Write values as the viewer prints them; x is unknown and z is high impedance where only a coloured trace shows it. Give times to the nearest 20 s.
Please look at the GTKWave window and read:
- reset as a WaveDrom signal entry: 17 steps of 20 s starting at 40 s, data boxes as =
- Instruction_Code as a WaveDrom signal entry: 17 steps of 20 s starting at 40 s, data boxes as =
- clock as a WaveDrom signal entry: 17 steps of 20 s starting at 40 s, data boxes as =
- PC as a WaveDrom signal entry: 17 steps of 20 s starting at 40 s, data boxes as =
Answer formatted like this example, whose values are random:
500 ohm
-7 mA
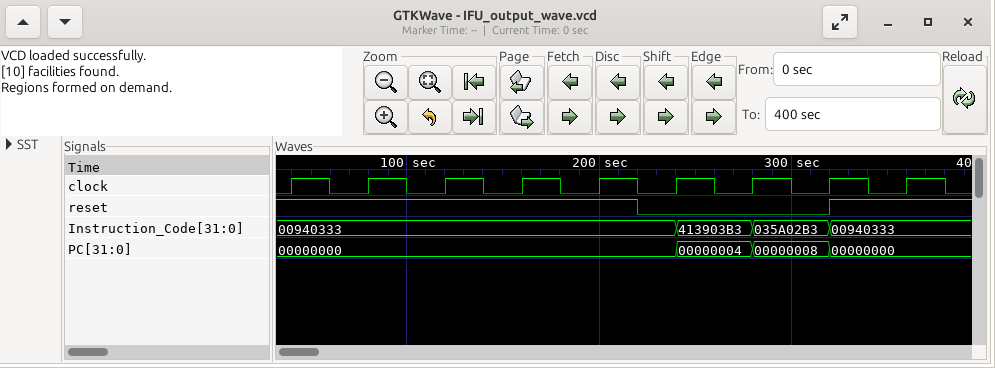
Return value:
{name: 'reset', wave: '1........0....1..'}
{name: 'Instruction_Code', wave: '=.........=.=.=..', data: '00940333 413903B3 035A02B3 00940333'}
{name: 'clock', wave: '10101010101010101'}
{name: 'PC', wave: '=.........=.=.=..', data: '00000000 00000004 00000008 00000000'}
